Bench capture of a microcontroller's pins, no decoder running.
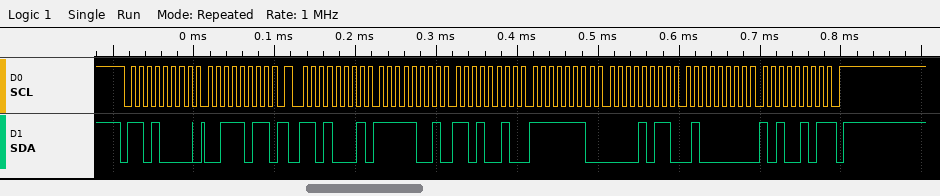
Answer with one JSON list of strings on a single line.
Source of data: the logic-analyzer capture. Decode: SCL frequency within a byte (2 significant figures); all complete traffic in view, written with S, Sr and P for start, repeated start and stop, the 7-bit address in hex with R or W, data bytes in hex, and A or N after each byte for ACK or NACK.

["100 kHz", "S 68W A 3B A Sr 68R A F9 A D2 A FE A 0B A 40 A A5 N P"]
